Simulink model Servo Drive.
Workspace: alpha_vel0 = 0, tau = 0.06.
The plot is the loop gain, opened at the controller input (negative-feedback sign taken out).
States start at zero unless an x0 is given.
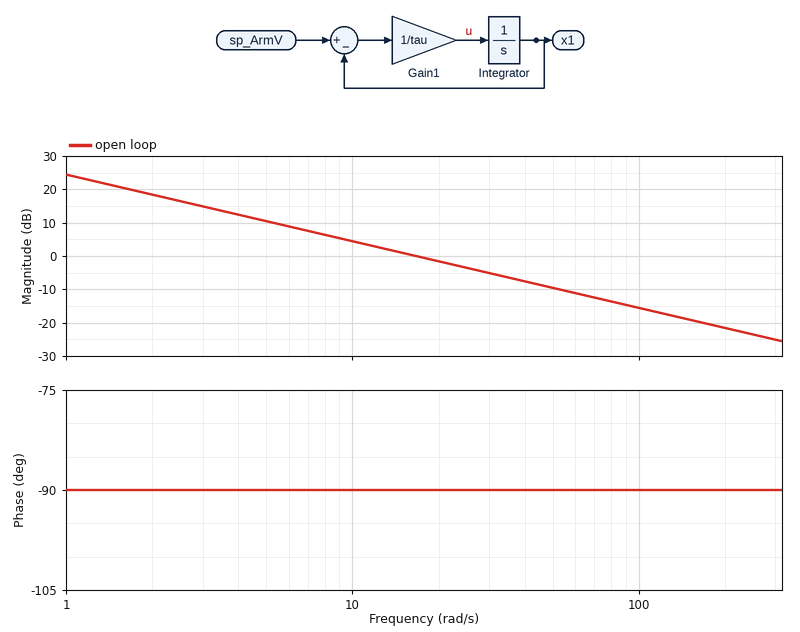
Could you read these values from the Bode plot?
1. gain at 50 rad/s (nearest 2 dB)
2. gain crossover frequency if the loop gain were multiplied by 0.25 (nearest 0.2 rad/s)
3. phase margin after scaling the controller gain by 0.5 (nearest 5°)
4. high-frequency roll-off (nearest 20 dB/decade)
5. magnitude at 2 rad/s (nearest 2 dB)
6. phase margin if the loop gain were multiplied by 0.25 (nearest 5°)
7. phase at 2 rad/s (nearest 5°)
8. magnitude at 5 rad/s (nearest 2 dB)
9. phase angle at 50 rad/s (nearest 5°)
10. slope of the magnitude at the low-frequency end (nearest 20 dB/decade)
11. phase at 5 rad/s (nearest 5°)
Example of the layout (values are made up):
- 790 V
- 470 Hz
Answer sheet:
- -10 dB
- 4.2 rad/s
- 90°
- -20 dB/decade
- 18 dB
- 90°
- -90°
- 10 dB
- -90°
- -20 dB/decade
- -90°
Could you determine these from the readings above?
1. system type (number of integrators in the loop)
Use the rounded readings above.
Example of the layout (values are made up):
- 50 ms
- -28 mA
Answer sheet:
- 1
